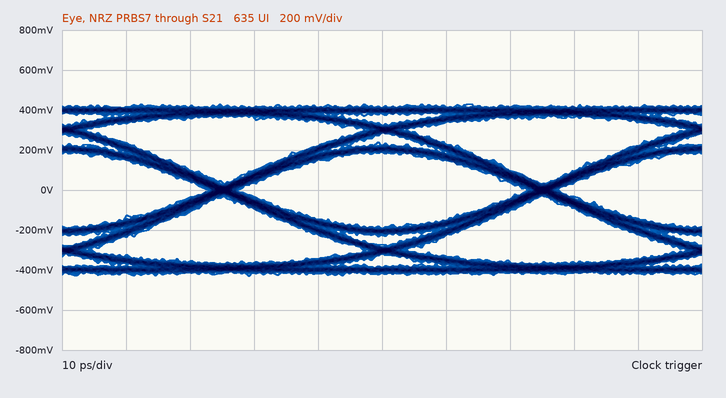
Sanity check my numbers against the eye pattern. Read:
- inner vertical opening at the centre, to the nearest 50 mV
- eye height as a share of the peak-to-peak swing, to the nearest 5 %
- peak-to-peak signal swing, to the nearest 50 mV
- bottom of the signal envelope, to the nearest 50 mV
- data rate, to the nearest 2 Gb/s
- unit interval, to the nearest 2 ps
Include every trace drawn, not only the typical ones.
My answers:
400 mV
45 %
850 mV
-450 mV
20 Gb/s
50 ps
